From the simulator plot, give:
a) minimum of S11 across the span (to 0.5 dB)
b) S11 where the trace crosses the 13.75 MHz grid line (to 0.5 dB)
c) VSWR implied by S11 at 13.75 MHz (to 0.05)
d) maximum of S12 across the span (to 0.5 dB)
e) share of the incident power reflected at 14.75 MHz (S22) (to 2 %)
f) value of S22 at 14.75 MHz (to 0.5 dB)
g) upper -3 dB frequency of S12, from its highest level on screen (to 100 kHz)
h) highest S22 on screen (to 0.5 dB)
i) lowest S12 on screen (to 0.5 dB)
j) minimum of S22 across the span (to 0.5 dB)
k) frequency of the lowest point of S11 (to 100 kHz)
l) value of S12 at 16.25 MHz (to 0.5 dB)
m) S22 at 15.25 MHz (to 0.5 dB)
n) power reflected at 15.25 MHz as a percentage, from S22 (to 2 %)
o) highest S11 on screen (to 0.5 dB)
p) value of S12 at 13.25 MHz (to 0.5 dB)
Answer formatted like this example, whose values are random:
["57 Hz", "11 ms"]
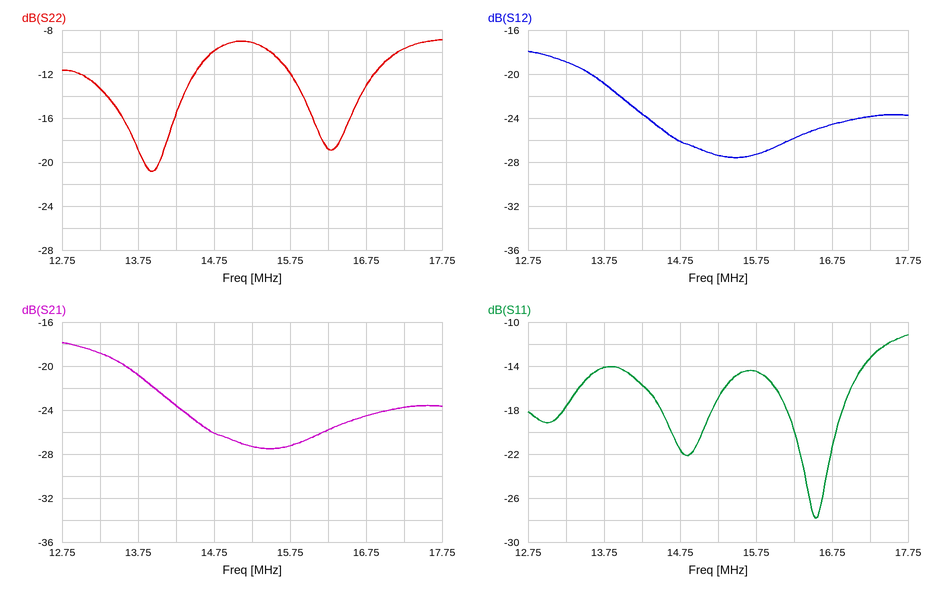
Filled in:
["-28.0 dB", "-14.0 dB", "1.50", "-18.0 dB", "10 %", "-10.0 dB", "13.8 MHz", "-9.0 dB", "-27.5 dB", "-21.0 dB", "16.5 MHz", "-26.0 dB", "-9.0 dB", "12 %", "-11.0 dB", "-19.0 dB"]
